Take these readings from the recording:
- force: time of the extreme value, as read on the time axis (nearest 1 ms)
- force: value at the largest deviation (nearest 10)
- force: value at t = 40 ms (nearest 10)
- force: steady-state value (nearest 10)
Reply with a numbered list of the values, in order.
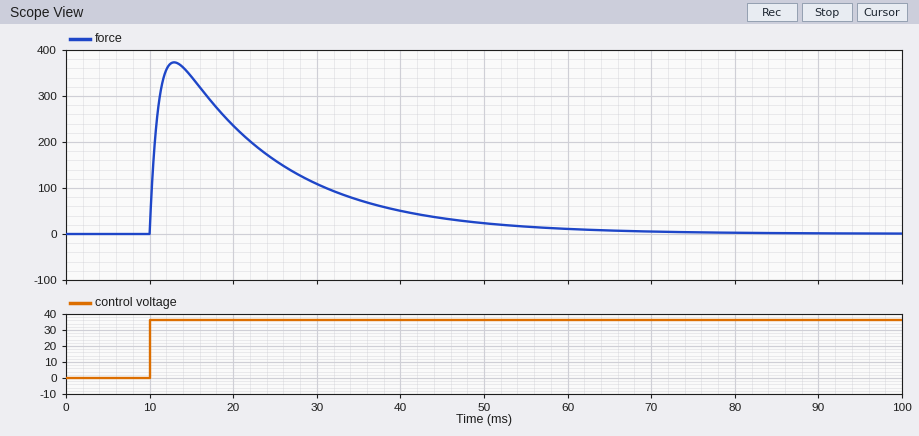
1. 13 ms
2. 370
3. 50
4. 0
